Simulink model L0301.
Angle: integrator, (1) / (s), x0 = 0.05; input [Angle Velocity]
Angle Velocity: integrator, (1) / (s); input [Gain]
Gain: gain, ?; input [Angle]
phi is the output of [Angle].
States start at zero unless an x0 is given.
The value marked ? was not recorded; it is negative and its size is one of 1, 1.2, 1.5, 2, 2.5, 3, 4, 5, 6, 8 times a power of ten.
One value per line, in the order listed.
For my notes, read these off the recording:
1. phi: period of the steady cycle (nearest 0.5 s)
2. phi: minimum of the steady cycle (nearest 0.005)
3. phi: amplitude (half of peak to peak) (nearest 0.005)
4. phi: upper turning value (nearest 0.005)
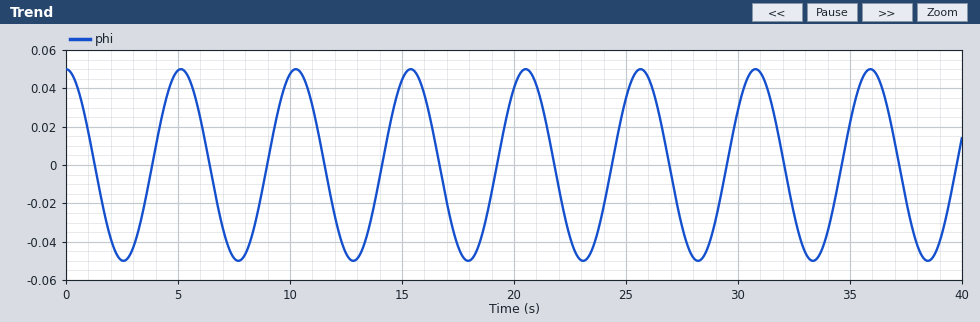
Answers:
5.0 s
-0.050
0.050
0.050
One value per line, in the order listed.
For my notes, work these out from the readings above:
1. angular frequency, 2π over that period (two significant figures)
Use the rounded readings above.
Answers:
1.3 rad/s
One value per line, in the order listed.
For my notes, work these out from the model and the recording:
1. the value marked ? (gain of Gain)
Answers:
-1.5
